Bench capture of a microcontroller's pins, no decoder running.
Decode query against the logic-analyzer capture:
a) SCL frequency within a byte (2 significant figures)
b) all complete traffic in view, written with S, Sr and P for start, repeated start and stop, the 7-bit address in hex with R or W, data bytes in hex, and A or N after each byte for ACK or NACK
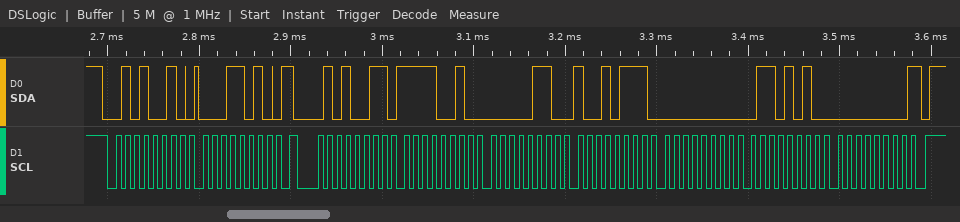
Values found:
100 kHz
S 29W A 1A A Sr 29R A F2 A 06 A 97 A 00 A 6A A 00 N P
